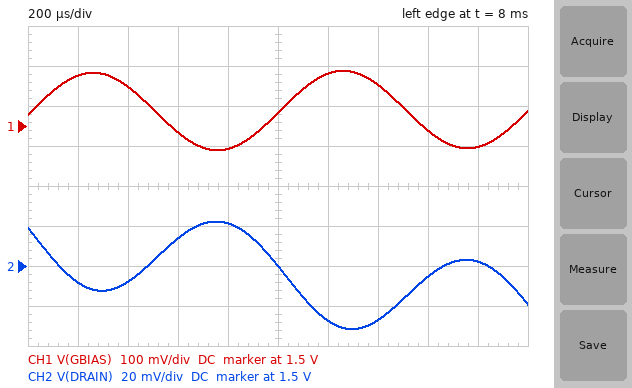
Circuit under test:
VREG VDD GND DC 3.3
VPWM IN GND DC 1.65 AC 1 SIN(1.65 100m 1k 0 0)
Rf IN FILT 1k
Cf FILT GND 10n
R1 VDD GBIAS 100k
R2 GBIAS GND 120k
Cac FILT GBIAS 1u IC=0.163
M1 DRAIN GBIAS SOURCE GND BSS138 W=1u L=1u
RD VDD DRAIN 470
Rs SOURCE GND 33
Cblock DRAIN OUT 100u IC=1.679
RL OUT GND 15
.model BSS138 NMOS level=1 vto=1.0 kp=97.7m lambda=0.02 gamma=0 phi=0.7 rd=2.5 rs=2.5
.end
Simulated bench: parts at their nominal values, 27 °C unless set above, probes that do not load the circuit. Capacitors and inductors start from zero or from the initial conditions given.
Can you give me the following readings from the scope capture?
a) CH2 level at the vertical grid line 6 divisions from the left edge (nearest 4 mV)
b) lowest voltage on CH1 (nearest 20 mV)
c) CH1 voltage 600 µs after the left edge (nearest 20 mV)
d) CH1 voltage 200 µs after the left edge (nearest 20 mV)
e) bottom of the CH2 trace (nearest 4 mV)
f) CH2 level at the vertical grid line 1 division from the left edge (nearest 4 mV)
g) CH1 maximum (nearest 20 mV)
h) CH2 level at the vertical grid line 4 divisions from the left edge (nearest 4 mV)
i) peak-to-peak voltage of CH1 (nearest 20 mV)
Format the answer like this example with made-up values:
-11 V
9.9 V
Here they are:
1.472 V
1.44 V
1.48 V
1.62 V
1.468 V
1.492 V
1.64 V
1.520 V
200 mV
